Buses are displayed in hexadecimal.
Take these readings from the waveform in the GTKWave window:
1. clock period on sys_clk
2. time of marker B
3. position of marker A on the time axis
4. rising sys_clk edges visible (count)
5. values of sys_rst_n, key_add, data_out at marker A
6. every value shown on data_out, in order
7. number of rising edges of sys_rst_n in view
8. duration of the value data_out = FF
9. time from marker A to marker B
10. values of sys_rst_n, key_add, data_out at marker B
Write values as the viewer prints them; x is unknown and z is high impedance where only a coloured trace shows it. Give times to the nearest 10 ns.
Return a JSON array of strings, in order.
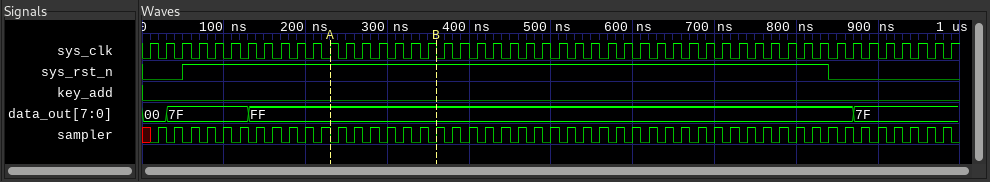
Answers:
["20 ns", "360 ns", "230 ns", "50", "sys_rst_n=1, key_add=0, data_out=FF", "00, 7F, FF, 7F", "1", "740 ns", "130 ns", "sys_rst_n=1, key_add=0, data_out=FF"]
